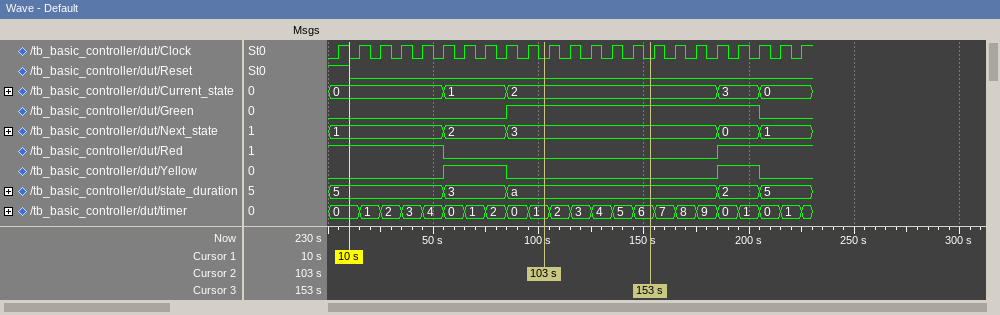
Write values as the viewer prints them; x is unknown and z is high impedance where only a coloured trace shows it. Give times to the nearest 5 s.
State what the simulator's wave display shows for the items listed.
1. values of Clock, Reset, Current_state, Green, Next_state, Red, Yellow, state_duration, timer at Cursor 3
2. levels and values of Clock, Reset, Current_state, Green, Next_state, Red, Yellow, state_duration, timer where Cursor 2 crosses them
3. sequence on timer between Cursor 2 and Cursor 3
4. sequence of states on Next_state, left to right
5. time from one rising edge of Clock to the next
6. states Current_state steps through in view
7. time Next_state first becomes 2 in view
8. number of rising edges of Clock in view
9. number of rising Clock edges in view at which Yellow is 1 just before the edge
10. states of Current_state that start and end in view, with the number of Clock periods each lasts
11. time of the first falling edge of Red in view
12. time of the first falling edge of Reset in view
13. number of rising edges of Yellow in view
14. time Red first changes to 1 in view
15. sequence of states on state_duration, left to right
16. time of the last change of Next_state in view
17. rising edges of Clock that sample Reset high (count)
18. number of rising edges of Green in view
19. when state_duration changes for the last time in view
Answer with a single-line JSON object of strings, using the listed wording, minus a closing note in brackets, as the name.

{"values of Clock, Reset, Current_state, Green, Next_state, Red, Yellow, state_duration, timer at Cursor 3": "Clock=0, Reset=0, Current_state=2, Green=1, Next_state=3, Red=0, Yellow=0, state_duration=a, timer=6", "levels and values of Clock, Reset, Current_state, Green, Next_state, Red, Yellow, state_duration, timer where Cursor 2 crosses them": "Clock=0, Reset=0, Current_state=2, Green=1, Next_state=3, Red=0, Yellow=0, state_duration=a, timer=1", "sequence on timer between Cursor 2 and Cursor 3": "1, 2, 3, 4, 5, 6", "sequence of states on Next_state, left to right": "1, 2, 3, 0, 1", "time from one rising edge of Clock to the next": "10 s", "states Current_state steps through in view": "0, 1, 2, 3, 0", "time Next_state first becomes 2 in view": "55 s", "number of rising edges of Clock in view": "23", "number of rising Clock edges in view at which Yellow is 1 just before the edge": "5", "states of Current_state that start and end in view, with the number of Clock periods each lasts": "1: 3, 2: 10, 3: 2", "time of the first falling edge of Red in view": "55 s", "time of the first falling edge of Reset in view": "10 s", "number of rising edges of Yellow in view": "2", "time Red first changes to 1 in view": "185 s", "sequence of states on state_duration, left to right": "5, 3, a, 2, 5", "time of the last change of Next_state in view": "205 s", "rising edges of Clock that sample Reset high": "1", "number of rising edges of Green in view": "1", "when state_duration changes for the last time in view": "205 s"}
